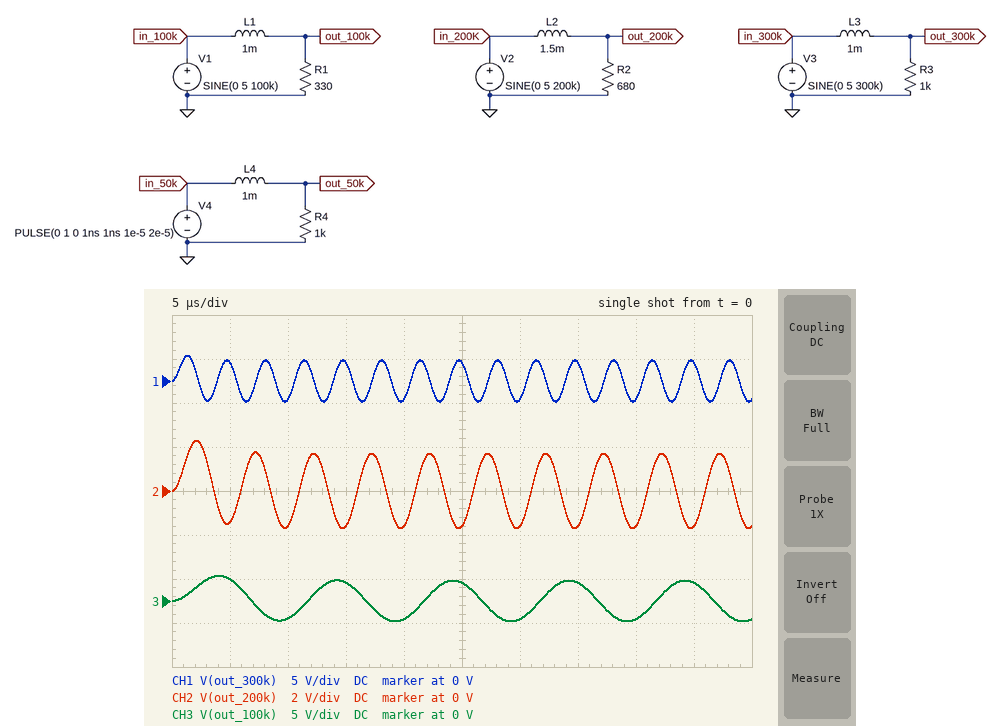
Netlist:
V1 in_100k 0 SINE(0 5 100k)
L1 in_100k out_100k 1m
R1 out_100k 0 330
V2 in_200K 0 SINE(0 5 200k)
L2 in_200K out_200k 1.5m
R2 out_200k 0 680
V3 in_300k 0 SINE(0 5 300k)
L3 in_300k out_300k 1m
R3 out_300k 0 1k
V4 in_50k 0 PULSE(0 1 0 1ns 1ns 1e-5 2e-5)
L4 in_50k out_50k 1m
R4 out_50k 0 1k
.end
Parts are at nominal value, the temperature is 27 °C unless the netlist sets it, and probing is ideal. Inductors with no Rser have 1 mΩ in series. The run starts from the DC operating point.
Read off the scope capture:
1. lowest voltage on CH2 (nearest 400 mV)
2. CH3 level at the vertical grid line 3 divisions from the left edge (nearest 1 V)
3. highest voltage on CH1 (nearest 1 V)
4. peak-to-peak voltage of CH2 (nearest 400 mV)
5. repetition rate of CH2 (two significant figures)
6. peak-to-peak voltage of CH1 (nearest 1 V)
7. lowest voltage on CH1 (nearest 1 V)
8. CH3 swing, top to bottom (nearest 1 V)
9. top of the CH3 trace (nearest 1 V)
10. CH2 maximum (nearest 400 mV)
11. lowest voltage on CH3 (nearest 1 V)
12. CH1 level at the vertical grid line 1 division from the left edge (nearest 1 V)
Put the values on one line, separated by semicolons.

-1.6 V; 2 V; 3 V; 4.0 V; 200 kHz; 5 V; -2 V; 5 V; 3 V; 2.4 V; -2 V; 2 V
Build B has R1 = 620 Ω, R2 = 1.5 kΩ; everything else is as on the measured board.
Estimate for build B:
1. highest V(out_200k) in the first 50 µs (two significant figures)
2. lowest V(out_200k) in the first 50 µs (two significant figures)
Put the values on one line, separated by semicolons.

3.5 V; -3.1 V
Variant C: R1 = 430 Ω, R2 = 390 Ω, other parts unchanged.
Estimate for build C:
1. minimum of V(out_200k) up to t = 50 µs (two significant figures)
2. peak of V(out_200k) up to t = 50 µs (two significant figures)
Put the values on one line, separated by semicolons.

-1.0 V; 1.6 V
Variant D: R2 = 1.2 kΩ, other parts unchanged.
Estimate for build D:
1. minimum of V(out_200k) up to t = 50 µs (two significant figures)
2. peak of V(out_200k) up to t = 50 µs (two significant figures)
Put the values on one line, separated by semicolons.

-2.7 V; 3.1 V
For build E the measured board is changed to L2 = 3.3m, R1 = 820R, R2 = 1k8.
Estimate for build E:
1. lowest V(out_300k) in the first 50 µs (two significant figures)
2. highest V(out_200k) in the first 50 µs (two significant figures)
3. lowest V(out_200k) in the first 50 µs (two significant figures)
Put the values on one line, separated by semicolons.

-2.3 V; 2.6 V; -2.0 V
